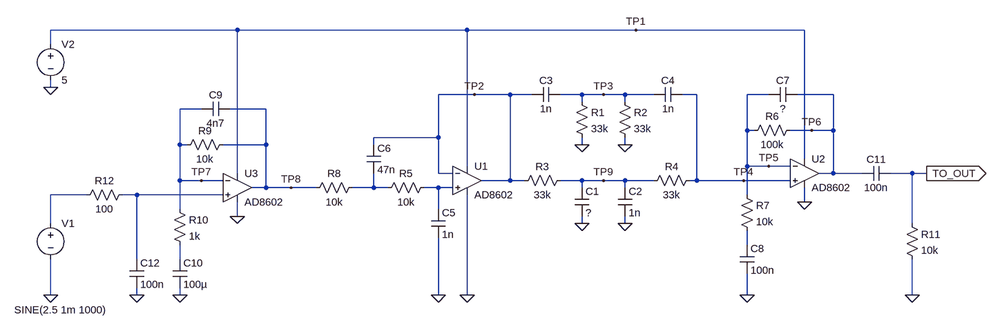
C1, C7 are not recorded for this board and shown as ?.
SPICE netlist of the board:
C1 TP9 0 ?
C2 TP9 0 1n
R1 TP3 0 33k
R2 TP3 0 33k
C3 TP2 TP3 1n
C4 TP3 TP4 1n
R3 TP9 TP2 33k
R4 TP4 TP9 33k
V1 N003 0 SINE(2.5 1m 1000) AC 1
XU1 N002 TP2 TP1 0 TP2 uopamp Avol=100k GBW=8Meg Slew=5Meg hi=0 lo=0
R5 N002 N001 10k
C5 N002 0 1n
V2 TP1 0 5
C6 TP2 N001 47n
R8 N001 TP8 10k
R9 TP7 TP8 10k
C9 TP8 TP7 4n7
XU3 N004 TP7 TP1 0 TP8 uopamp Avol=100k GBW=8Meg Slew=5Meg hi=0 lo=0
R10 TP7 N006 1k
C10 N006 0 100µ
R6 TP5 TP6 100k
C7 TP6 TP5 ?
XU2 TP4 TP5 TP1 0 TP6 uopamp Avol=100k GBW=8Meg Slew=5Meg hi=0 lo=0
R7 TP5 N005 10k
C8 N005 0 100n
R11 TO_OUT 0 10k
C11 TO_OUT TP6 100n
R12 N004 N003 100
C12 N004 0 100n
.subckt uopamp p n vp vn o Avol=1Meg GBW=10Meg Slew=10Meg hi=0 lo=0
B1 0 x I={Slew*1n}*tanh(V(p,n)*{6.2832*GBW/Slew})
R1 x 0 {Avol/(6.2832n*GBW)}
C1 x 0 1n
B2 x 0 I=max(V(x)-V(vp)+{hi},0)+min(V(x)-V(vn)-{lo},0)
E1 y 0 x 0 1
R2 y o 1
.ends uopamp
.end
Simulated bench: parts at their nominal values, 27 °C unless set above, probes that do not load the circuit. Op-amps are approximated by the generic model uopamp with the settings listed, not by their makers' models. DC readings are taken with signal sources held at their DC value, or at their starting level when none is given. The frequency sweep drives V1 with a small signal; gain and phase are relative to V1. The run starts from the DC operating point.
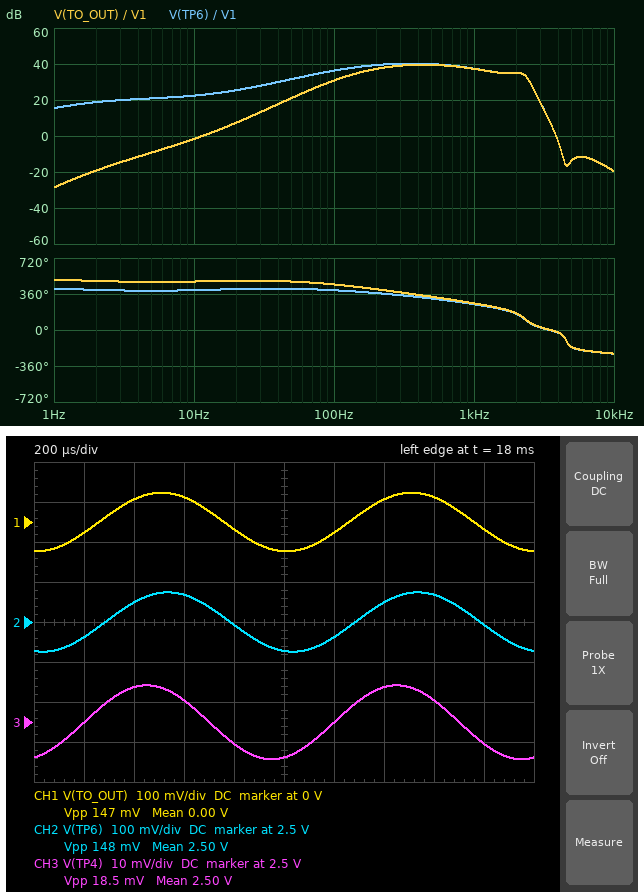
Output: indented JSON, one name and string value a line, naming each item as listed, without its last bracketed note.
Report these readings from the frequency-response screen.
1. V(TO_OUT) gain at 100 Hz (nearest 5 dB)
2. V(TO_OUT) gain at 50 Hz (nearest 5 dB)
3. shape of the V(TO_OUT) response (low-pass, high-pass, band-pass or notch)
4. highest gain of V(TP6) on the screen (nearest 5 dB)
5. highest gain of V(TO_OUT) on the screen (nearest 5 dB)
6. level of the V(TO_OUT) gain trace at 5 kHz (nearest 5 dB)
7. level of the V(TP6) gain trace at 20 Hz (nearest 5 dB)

{
  "V(TO_OUT) gain at 100 Hz": "30 dB",
  "V(TO_OUT) gain at 50 Hz": "20 dB",
  "shape of the V(TO_OUT) response": "band-pass",
  "highest gain of V(TP6) on the screen": "40 dB",
  "highest gain of V(TO_OUT) on the screen": "40 dB",
  "level of the V(TO_OUT) gain trace at 5 kHz": "-15 dB",
  "level of the V(TP6) gain trace at 20 Hz": "25 dB"
}
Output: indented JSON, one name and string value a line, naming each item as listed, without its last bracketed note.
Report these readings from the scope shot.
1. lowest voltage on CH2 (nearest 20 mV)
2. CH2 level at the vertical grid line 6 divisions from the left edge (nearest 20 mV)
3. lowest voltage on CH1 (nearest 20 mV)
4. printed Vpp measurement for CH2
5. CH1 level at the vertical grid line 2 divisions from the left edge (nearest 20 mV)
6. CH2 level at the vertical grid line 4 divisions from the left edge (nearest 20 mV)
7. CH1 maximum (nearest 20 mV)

{
  "lowest voltage on CH2": "2.42 V",
  "CH2 level at the vertical grid line 6 divisions from the left edge": "2.46 V",
  "lowest voltage on CH1": "-80 mV",
  "printed Vpp measurement for CH2": "148 mV",
  "CH1 level at the vertical grid line 2 divisions from the left edge": "60 mV",
  "CH2 level at the vertical grid line 4 divisions from the left edge": "2.50 V",
  "CH1 maximum": "80 mV"
}
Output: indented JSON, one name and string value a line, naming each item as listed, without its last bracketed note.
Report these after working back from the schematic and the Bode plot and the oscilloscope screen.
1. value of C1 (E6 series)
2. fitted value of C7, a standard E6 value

{
  "value of C1": "1.5 nF",
  "fitted value of C7, a standard E6 value": "1.5 nF"
}
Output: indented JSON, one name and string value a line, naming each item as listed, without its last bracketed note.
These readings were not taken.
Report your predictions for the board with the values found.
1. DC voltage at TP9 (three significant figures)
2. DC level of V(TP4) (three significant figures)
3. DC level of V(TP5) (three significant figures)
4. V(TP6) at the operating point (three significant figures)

{
  "DC voltage at TP9": "2.50 V",
  "DC level of V(TP4)": "2.50 V",
  "DC level of V(TP5)": "2.50 V",
  "V(TP6) at the operating point": "2.50 V"
}
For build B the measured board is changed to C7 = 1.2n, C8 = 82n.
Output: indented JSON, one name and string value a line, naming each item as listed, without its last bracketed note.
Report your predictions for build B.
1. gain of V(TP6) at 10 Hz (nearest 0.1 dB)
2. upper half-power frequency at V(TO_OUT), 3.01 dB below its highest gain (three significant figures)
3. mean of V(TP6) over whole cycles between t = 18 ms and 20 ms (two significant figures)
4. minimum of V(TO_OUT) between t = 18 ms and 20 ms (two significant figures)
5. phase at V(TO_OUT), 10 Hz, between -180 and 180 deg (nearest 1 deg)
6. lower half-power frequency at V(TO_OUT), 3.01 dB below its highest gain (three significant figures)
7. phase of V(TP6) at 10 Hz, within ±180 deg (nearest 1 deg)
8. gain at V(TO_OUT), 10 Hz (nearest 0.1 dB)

{
  "gain of V(TP6) at 10 Hz": "21.9 dB",
  "upper half-power frequency at V(TO_OUT), 3.01 dB below its highest gain": "1.38 kHz",
  "mean of V(TP6) over whole cycles between t = 18 ms and 20 ms": "2.5 V",
  "minimum of V(TO_OUT) between t = 18 ms and 20 ms": "-80 mV",
  "phase at V(TO_OUT), 10 Hz, between -180 and 180 deg": "120 deg",
  "lower half-power frequency at V(TO_OUT), 3.01 dB below its highest gain": "201 Hz",
  "phase of V(TP6) at 10 Hz, within ±180 deg": "34 deg",
  "gain at V(TO_OUT), 10 Hz": "-2.1 dB"
}
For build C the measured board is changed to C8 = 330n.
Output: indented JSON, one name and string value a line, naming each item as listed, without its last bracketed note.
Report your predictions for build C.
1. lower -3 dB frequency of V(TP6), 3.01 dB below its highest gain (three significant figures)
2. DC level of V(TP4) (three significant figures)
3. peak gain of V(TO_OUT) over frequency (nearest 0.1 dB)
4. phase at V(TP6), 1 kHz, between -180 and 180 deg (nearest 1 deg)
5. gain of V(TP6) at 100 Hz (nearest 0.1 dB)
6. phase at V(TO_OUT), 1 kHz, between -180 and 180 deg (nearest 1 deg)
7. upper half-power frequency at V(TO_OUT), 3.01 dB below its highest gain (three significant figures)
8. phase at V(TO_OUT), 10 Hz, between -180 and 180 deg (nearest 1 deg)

{
  "lower -3 dB frequency of V(TP6), 3.01 dB below its highest gain": "43.1 Hz",
  "DC level of V(TP4)": "2.50 V",
  "peak gain of V(TO_OUT) over frequency": "40.1 dB",
  "phase at V(TP6), 1 kHz, between -180 and 180 deg": "-108 deg",
  "gain of V(TP6) at 100 Hz": "40.7 dB",
  "phase at V(TO_OUT), 1 kHz, between -180 and 180 deg": "-99 deg",
  "upper half-power frequency at V(TO_OUT), 3.01 dB below its highest gain": "1.05 kHz",
  "phase at V(TO_OUT), 10 Hz, between -180 and 180 deg": "148 deg"
}
